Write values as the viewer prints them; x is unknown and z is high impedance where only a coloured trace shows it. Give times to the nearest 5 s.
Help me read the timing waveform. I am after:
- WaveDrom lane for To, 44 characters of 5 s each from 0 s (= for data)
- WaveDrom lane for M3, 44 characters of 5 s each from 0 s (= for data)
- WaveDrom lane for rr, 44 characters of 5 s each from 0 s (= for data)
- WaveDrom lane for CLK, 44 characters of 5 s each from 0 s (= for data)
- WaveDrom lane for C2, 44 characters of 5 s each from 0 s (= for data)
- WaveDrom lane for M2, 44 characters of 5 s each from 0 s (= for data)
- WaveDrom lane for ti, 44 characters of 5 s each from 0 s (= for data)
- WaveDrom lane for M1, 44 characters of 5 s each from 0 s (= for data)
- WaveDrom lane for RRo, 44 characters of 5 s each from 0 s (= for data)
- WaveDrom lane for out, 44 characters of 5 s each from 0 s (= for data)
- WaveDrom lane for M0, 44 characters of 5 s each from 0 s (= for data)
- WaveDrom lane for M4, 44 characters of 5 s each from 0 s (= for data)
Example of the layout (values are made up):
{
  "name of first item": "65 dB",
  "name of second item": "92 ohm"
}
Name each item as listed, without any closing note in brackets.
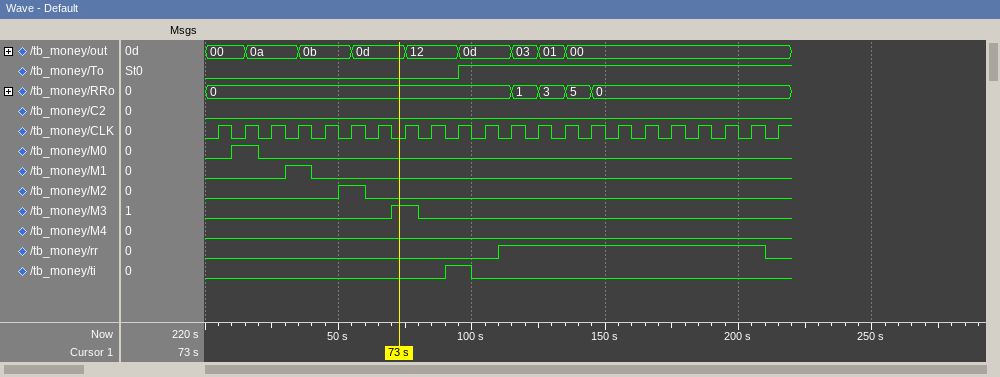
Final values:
{
  "WaveDrom lane for To, 44 characters of 5 s each from 0 s": "{name: 'To', wave: '0..................1........................'}",
  "WaveDrom lane for M3, 44 characters of 5 s each from 0 s": "{name: 'M3', wave: '0.............1.0...........................'}",
  "WaveDrom lane for rr, 44 characters of 5 s each from 0 s": "{name: 'rr', wave: '0.....................1...................0.'}",
  "WaveDrom lane for CLK, 44 characters of 5 s each from 0 s": "{name: 'CLK', wave: '01010101010101010101010101010101010101010101'}",
  "WaveDrom lane for C2, 44 characters of 5 s each from 0 s": "{name: 'C2', wave: '0...........................................'}",
  "WaveDrom lane for M2, 44 characters of 5 s each from 0 s": "{name: 'M2', wave: '0.........1.0...............................'}",
  "WaveDrom lane for ti, 44 characters of 5 s each from 0 s": "{name: 'ti', wave: '0.................1.0.......................'}",
  "WaveDrom lane for M1, 44 characters of 5 s each from 0 s": "{name: 'M1', wave: '0.....1.0...................................'}",
  "WaveDrom lane for RRo, 44 characters of 5 s each from 0 s": "{name: 'RRo', wave: '=......................=.=.=.=..............', data: '0 1 3 5 0'}",
  "WaveDrom lane for out, 44 characters of 5 s each from 0 s": "{name: 'out', wave: '=..=...=...=...=...=...=.=.=................', data: '00 0a 0b 0d 12 0d 03 01 00'}",
  "WaveDrom lane for M0, 44 characters of 5 s each from 0 s": "{name: 'M0', wave: '0.1.0.......................................'}",
  "WaveDrom lane for M4, 44 characters of 5 s each from 0 s": "{name: 'M4', wave: '0...........................................'}"
}
